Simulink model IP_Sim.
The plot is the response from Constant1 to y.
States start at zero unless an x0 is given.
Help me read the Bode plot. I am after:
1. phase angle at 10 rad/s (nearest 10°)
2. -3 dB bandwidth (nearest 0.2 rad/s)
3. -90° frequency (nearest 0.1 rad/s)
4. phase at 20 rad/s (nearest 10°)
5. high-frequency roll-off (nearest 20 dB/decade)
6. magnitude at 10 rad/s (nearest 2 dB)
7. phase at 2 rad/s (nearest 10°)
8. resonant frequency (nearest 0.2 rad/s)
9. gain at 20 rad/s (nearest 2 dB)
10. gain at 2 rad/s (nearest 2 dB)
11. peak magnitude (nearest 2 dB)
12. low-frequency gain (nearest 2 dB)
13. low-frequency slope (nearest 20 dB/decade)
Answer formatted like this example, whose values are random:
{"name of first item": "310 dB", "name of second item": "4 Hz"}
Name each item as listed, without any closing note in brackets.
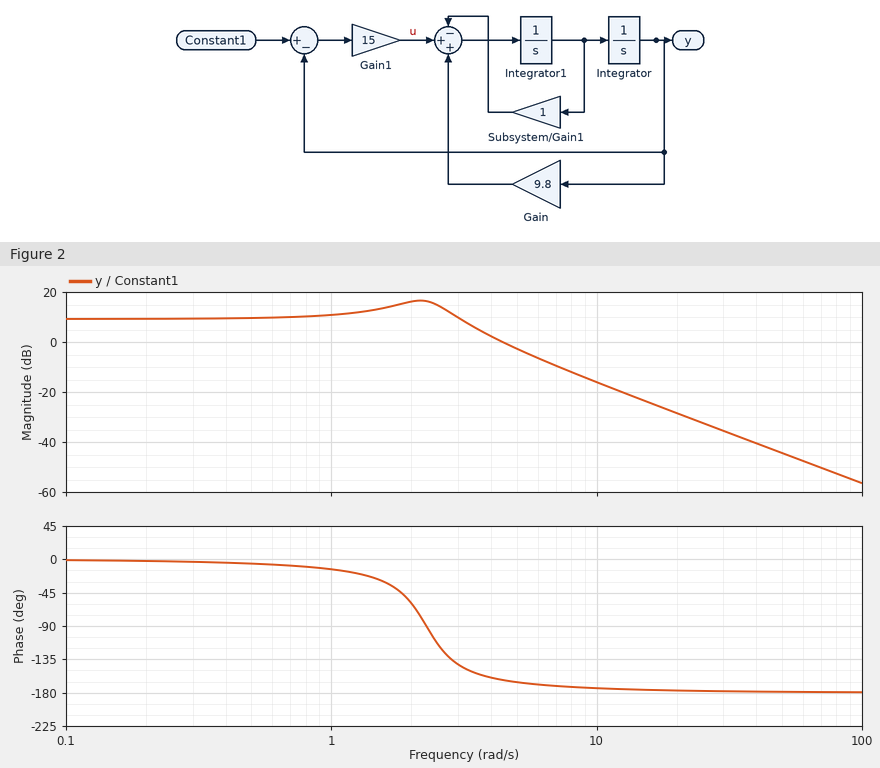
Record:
{"phase angle at 10 rad/s": "-170°", "-3 dB bandwidth": "3.4 rad/s", "-90° frequency": "2.3 rad/s", "phase at 20 rad/s": "-180°", "high-frequency roll-off": "-40 dB/decade", "magnitude at 10 rad/s": "-16 dB", "phase at 2 rad/s": "-60°", "resonant frequency": "2.2 rad/s", "gain at 20 rad/s": "-28 dB", "gain at 2 rad/s": "16 dB", "peak magnitude": "16 dB", "low-frequency gain": "10 dB", "low-frequency slope": "0 dB/decade"}
